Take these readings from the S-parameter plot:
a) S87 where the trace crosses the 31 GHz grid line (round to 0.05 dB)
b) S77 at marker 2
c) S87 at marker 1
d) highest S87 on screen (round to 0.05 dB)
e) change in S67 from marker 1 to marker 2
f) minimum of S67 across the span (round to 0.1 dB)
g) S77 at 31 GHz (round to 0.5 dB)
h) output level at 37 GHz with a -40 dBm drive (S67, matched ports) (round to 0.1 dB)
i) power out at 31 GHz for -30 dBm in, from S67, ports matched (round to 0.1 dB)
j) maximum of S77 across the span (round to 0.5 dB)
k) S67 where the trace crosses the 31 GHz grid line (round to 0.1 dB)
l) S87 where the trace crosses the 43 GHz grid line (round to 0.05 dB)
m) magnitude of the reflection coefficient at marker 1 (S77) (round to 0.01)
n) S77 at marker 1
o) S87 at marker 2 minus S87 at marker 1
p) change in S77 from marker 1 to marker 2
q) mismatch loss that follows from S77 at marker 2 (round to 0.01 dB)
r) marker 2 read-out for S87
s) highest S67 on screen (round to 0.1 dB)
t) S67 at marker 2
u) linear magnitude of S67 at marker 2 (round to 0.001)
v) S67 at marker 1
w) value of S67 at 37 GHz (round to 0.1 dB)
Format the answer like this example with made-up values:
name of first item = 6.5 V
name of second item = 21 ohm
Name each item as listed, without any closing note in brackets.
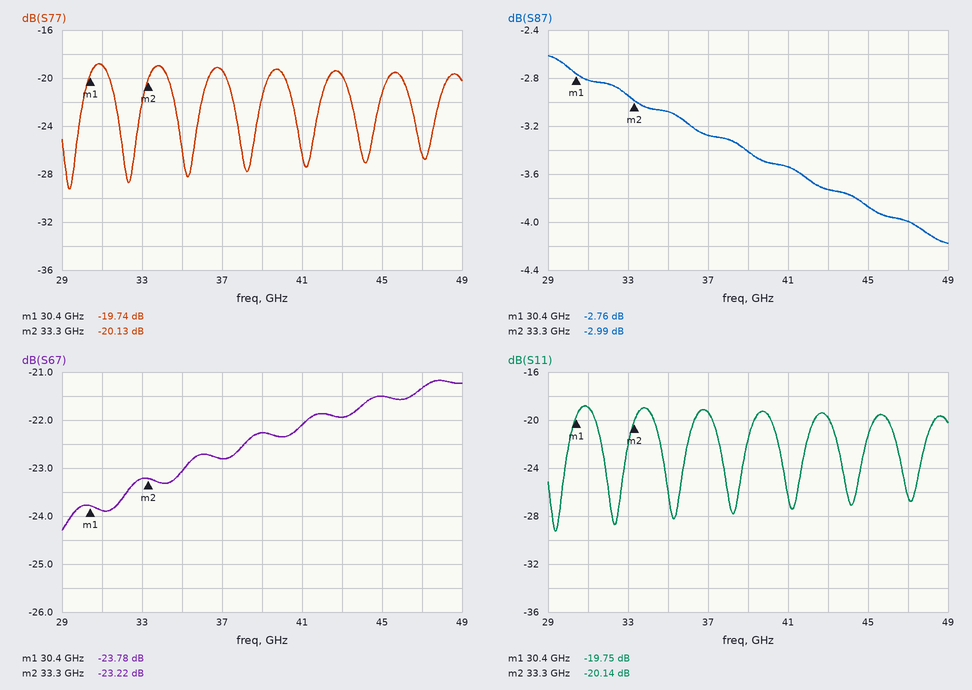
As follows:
S87 where the trace crosses the 31 GHz grid line = -2.80 dB
S77 at marker 2 = -20.13 dB
S87 at marker 1 = -2.76 dB
highest S87 on screen = -2.60 dB
change in S67 from marker 1 to marker 2 = 0.56 dB
minimum of S67 across the span = -24.3 dB
S77 at 31 GHz = -19.0 dB
output level at 37 GHz with a -40 dBm drive (S67, matched ports) = -62.8 dBm
power out at 31 GHz for -30 dBm in, from S67, ports matched = -53.9 dBm
maximum of S77 across the span = -19.0 dB
S67 where the trace crosses the 31 GHz grid line = -23.9 dB
S87 where the trace crosses the 43 GHz grid line = -3.75 dB
magnitude of the reflection coefficient at marker 1 (S77) = 0.10
S77 at marker 1 = -19.74 dB
S87 at marker 2 minus S87 at marker 1 = -0.23 dB
change in S77 from marker 1 to marker 2 = -0.39 dB
mismatch loss that follows from S77 at marker 2 = 0.04 dB
marker 2 read-out for S87 = -2.99 dB
highest S67 on screen = -21.2 dB
S67 at marker 2 = -23.22 dB
linear magnitude of S67 at marker 2 = 0.069
S67 at marker 1 = -23.78 dB
value of S67 at 37 GHz = -22.8 dB
